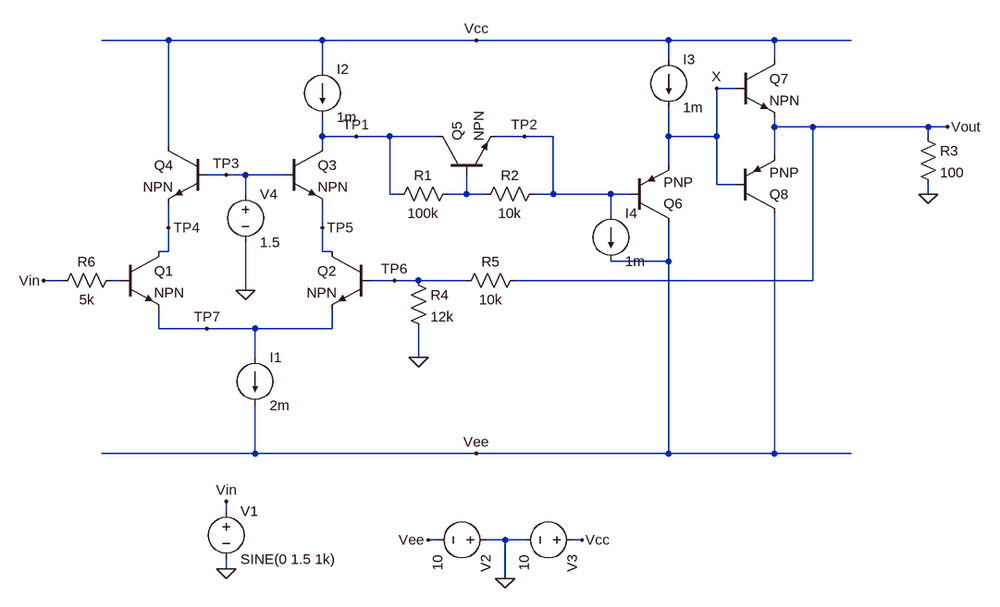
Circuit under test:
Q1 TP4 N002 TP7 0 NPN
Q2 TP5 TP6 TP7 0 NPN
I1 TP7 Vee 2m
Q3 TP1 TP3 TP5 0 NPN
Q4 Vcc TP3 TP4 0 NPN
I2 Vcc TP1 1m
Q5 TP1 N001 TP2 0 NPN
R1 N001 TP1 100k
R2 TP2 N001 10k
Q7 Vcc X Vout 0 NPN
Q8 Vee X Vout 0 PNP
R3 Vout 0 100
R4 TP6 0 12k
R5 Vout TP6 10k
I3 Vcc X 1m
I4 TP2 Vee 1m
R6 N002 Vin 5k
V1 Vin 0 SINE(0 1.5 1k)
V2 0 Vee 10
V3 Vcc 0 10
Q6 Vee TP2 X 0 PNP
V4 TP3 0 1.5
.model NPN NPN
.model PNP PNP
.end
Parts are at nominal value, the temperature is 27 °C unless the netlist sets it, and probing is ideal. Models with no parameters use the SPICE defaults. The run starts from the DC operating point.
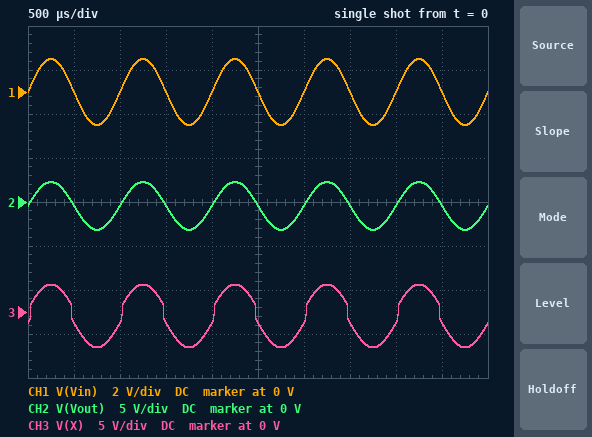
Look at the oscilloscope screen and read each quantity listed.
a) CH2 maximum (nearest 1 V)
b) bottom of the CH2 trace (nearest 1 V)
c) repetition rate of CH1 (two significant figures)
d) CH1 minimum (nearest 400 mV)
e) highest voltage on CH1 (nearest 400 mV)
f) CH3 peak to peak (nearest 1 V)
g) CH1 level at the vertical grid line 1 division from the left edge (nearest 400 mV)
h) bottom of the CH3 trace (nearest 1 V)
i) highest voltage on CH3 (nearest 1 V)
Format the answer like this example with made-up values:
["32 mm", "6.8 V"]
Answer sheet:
["2 V", "-3 V", "1.0 kHz", "-1.6 V", "1.6 V", "7 V", "0 V", "-4 V", "3 V"]
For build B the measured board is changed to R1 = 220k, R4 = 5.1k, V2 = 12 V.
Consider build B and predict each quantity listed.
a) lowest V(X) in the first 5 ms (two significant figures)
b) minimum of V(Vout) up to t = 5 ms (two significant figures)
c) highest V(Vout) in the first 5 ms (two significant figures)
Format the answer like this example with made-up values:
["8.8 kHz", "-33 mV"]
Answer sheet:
["-6.0 V", "-5.1 V", "3.6 V"]
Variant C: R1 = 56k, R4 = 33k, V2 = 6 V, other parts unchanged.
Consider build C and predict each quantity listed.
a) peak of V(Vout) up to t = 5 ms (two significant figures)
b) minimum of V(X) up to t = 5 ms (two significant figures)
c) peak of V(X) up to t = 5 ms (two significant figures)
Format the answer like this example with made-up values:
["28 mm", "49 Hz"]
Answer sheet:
["1.6 V", "-3.1 V", "2.4 V"]
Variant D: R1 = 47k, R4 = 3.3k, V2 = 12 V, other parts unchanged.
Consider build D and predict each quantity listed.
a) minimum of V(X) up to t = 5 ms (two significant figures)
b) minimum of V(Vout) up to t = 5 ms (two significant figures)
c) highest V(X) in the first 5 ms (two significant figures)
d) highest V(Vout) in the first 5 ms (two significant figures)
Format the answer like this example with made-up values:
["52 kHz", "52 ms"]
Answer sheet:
["-3.3 V", "-2.5 V", "5.7 V", "4.9 V"]
